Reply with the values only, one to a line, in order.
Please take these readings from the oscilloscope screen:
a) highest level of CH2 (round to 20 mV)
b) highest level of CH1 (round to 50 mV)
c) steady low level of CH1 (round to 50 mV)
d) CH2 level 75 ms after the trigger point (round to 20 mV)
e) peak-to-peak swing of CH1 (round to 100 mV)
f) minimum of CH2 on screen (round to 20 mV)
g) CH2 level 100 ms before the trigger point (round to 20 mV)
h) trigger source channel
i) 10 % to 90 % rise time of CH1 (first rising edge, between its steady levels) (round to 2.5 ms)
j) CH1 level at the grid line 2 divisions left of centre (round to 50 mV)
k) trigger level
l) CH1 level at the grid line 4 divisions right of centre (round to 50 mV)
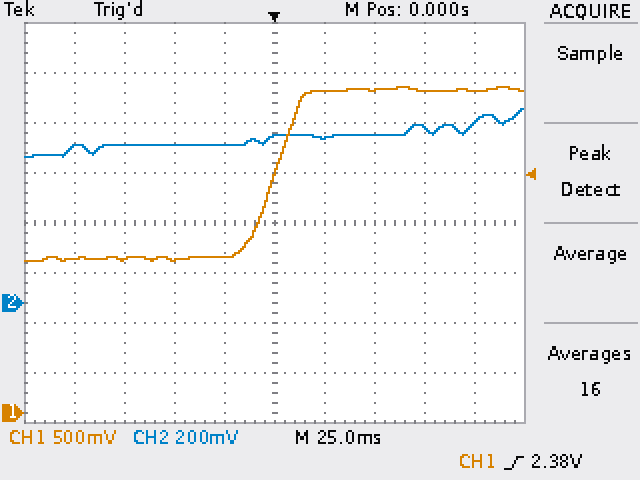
780 mV
3.25 V
1.55 V
700 mV
1.70 V
580 mV
620 mV
CH1
25.0 ms
1.55 V
2.38 V
3.20 V
